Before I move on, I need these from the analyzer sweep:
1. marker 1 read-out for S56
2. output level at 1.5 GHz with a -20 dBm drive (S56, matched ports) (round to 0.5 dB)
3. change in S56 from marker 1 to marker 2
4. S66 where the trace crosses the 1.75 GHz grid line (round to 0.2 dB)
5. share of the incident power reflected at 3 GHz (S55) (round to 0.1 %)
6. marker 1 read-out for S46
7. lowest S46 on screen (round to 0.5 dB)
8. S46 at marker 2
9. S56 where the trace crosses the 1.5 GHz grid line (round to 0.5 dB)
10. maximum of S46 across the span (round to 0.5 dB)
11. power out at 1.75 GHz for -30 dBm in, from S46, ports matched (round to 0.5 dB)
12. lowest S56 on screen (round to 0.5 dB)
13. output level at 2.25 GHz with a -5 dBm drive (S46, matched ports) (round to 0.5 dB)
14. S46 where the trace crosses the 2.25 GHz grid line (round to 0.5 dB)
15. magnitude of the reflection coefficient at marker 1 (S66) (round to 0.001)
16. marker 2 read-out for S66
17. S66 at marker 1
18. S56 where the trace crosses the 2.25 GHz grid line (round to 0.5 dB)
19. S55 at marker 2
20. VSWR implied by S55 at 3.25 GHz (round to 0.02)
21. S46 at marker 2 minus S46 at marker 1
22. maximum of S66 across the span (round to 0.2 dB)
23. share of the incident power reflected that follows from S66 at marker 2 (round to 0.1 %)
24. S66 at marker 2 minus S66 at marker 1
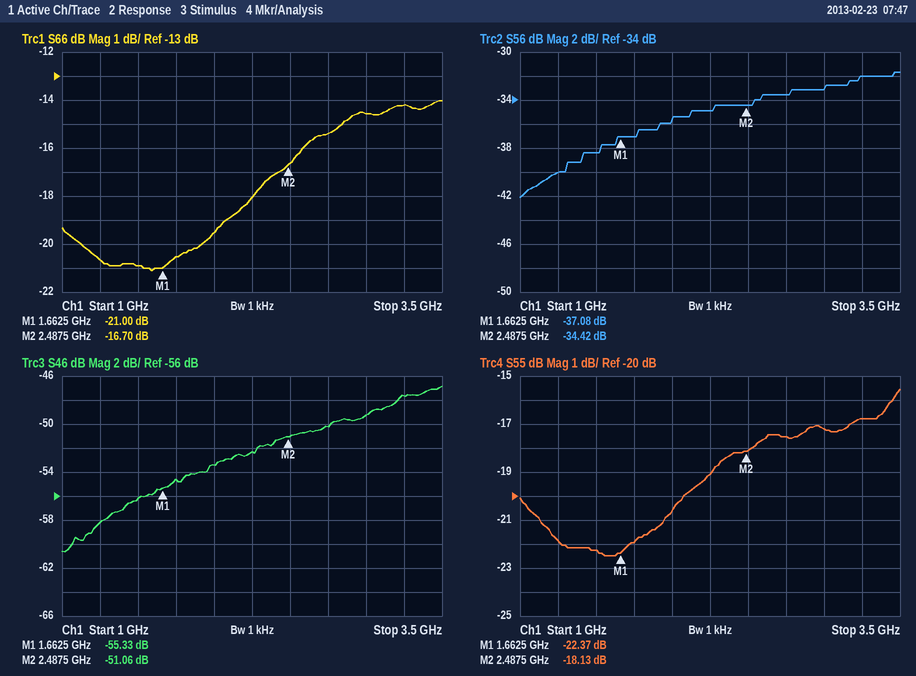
-37.08 dB
-58.5 dBm
2.66 dB
-20.6 dB
1.9 %
-55.33 dB
-60.5 dB
-51.06 dB
-38.5 dB
-47.0 dB
-84.5 dBm
-42.0 dB
-57.5 dBm
-52.5 dB
0.089
-16.70 dB
-21.00 dB
-35.0 dB
-18.13 dB
1.34
4.27 dB
-14.0 dB
2.1 %
4.30 dB
